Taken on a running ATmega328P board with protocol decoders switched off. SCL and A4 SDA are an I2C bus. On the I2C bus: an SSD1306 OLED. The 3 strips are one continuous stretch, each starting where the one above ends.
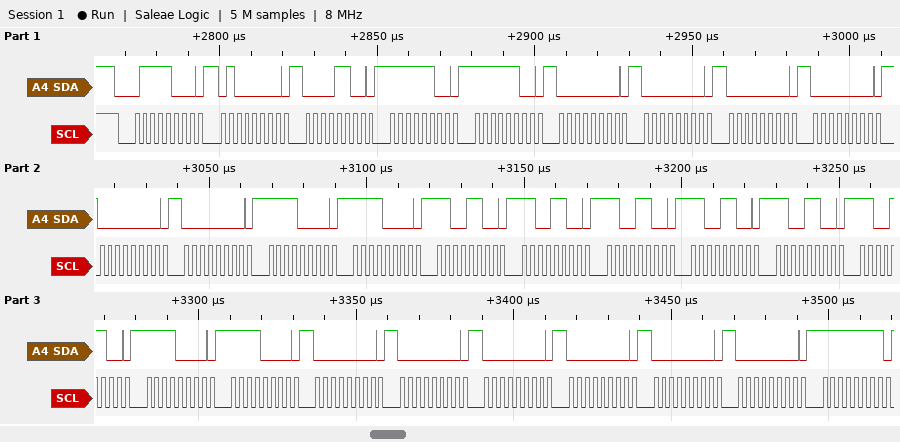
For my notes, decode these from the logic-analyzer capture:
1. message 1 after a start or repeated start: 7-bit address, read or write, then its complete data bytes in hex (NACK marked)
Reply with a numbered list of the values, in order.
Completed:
1. 0x3C write: 40 0C FC FC 00 00 00 00 00 00 F0 F0 CC CC CC CC CC CC F0 F0 00 00 00 00 00 00 FF
